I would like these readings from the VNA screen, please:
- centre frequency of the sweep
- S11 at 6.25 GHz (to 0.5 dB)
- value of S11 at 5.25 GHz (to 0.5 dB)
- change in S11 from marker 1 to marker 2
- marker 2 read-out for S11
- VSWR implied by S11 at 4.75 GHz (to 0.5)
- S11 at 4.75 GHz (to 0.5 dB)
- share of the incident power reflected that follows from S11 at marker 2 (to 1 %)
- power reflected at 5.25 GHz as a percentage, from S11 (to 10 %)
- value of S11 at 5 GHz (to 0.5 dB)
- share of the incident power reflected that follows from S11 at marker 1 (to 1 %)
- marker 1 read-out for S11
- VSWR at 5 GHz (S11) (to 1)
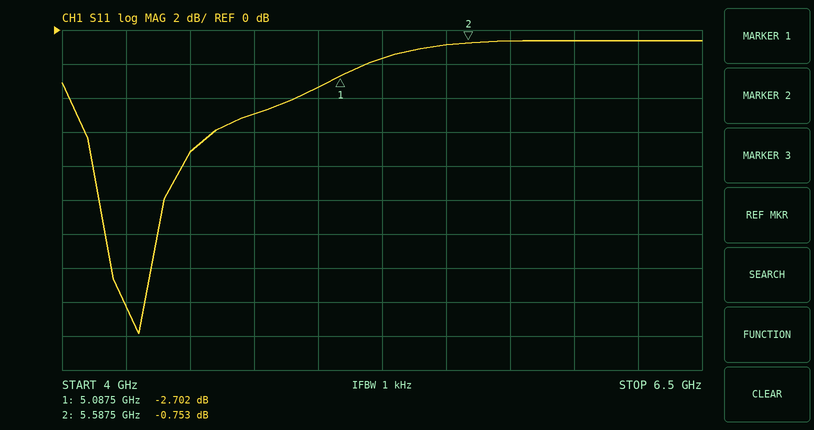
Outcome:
5.25 GHz
-0.5 dB
-1.5 dB
1.949 dB
-0.753 dB
3.5
-5.0 dB
84 %
70 %
-3.5 dB
54 %
-2.702 dB
5
